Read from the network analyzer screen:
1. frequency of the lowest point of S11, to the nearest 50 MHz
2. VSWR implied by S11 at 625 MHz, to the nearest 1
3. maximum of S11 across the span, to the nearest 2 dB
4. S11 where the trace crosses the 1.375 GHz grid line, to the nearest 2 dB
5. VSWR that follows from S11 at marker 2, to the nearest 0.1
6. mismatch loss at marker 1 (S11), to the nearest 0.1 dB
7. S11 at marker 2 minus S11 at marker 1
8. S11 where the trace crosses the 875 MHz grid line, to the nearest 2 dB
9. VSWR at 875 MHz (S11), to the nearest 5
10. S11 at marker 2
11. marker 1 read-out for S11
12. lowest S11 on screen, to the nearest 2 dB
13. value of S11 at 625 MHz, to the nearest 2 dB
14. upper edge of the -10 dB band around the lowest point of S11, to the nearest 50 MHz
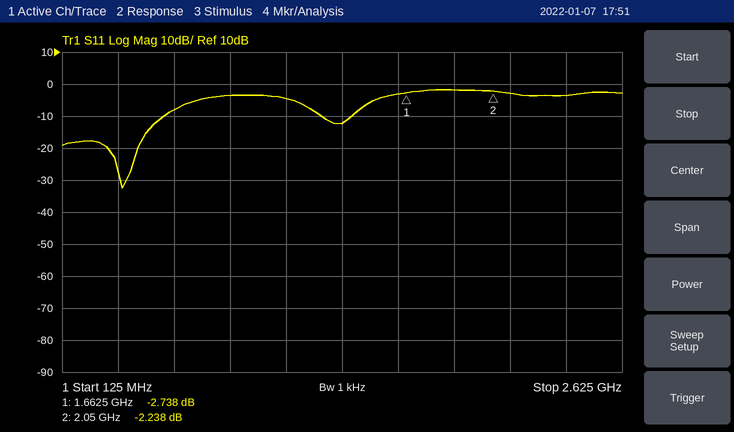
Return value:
400 MHz
2
-2 dB
-12 dB
7.8
3.3 dB
0.500 dB
-4 dB
5
-2.238 dB
-2.738 dB
-32 dB
-8 dB
600 MHz
